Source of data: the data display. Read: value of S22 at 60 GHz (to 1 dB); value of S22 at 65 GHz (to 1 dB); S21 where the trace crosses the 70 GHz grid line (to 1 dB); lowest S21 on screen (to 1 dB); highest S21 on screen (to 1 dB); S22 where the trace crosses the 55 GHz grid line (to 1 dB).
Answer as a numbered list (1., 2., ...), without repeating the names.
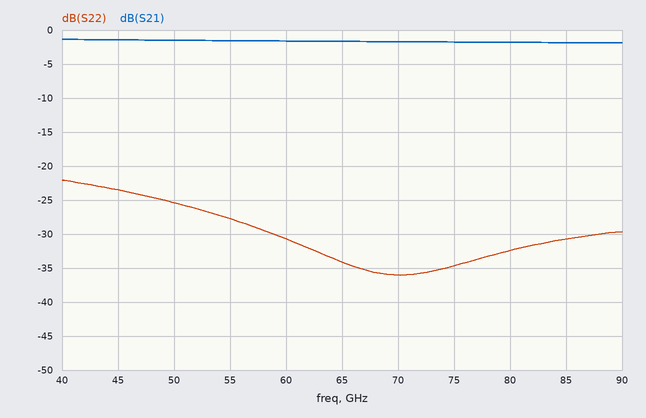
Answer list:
1. -31 dB
2. -34 dB
3. -2 dB
4. -2 dB
5. -1 dB
6. -28 dB
